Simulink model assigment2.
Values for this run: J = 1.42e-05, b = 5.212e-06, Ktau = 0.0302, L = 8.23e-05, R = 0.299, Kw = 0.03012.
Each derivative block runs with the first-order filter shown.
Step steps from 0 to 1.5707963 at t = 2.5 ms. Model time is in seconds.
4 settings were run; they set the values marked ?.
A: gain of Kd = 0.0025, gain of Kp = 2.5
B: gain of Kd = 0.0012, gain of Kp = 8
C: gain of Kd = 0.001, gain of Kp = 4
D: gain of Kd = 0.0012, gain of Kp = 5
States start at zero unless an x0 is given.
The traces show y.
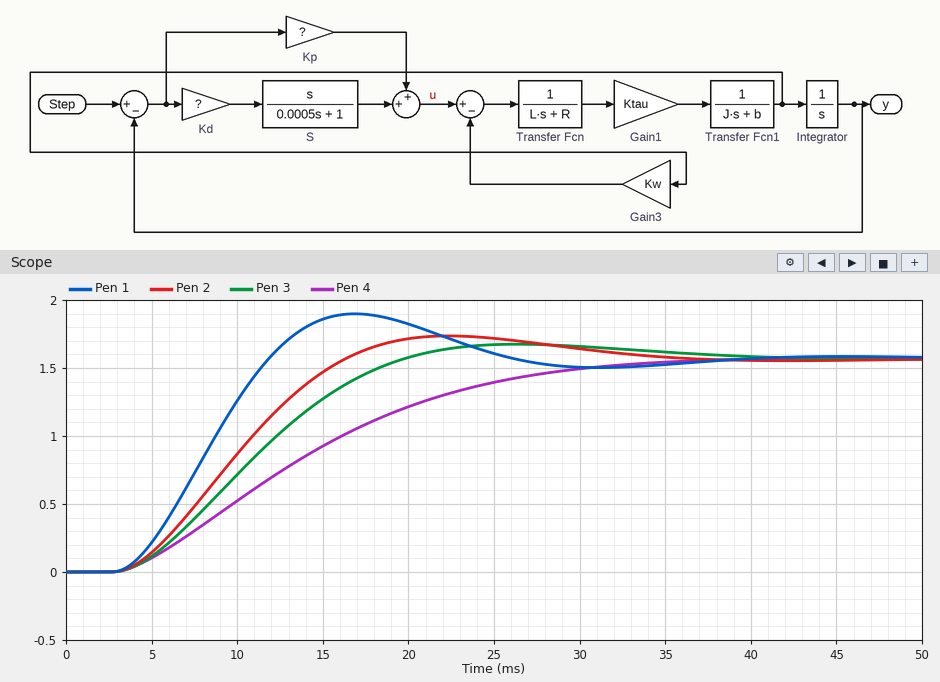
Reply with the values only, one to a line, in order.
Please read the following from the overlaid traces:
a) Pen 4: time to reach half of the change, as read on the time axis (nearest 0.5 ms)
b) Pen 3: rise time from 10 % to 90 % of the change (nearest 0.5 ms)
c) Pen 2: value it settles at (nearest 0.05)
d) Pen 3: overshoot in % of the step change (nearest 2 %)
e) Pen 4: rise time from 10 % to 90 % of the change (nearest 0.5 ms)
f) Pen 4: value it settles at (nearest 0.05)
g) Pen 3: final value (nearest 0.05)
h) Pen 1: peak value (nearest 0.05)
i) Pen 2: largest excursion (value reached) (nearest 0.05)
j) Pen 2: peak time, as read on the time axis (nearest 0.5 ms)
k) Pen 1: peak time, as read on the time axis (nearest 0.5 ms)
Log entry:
13.0 ms
11.5 ms
1.55
6 %
20.0 ms
1.55
1.55
1.90
1.75
22.5 ms
17.0 ms
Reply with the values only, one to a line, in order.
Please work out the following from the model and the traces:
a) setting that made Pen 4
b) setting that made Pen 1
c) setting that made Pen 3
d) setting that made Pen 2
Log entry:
A
B
C
D
